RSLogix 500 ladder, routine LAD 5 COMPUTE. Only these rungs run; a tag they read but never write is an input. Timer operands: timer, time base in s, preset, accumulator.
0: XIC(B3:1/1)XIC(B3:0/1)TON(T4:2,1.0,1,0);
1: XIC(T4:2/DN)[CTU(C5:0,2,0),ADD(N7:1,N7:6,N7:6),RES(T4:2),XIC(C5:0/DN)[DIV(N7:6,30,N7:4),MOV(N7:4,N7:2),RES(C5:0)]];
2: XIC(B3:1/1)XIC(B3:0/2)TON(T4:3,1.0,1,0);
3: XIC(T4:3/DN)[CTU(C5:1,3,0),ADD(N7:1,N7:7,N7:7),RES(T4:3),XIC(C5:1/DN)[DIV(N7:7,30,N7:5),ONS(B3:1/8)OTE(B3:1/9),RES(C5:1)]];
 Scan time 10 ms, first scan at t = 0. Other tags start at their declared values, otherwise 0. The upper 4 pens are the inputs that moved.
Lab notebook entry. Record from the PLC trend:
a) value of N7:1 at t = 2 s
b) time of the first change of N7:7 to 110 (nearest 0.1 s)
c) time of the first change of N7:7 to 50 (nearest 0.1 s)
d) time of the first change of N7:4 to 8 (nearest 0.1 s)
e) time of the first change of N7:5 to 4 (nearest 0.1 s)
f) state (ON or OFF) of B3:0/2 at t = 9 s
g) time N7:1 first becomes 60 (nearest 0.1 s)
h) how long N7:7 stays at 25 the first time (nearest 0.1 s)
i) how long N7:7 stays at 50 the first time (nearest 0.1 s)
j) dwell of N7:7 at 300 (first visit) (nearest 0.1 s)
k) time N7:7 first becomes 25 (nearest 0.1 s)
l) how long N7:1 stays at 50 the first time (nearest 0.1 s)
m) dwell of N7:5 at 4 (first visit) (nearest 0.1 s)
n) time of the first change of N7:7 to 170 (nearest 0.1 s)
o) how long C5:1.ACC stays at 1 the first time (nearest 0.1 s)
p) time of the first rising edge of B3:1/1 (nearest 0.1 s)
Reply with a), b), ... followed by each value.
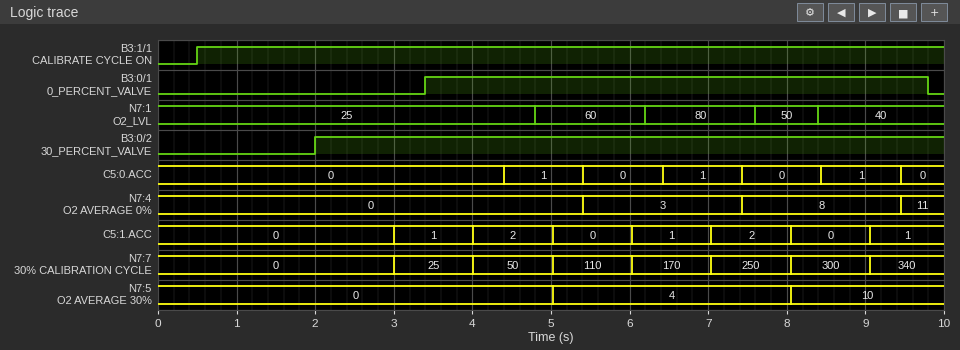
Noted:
a) 25
b) 5.0 s
c) 4.0 s
d) 7.4 s
e) 5.0 s
f) ON
g) 4.8 s
h) 1.0 s
i) 1.0 s
j) 1.0 s
k) 3.0 s
l) 0.8 s
m) 3.0 s
n) 6.0 s
o) 1.0 s
p) 0.5 s
